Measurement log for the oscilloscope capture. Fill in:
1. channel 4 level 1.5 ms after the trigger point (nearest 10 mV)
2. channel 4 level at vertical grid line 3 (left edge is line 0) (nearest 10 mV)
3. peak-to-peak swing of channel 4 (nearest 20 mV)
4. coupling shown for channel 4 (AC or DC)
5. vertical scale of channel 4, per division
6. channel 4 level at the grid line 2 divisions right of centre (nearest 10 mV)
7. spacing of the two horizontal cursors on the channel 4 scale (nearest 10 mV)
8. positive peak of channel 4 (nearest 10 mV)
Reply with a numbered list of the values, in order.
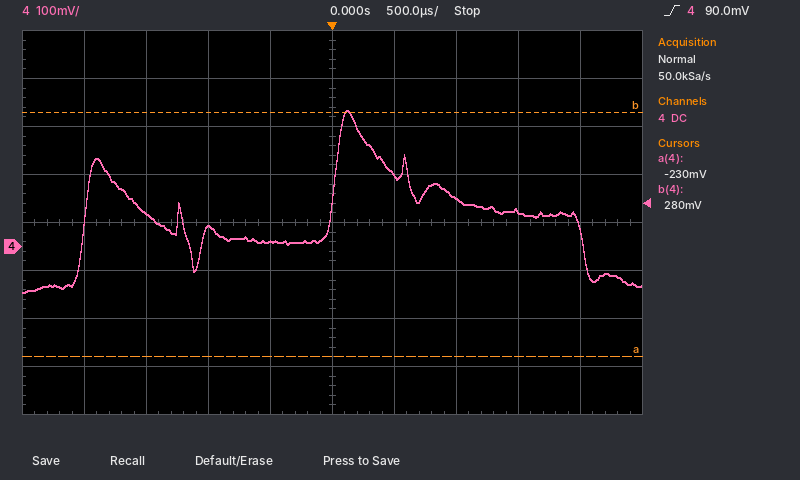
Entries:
1. 70 mV
2. 40 mV
3. 380 mV
4. DC
5. 100 mV
6. 100 mV
7. 510 mV
8. 280 mV
